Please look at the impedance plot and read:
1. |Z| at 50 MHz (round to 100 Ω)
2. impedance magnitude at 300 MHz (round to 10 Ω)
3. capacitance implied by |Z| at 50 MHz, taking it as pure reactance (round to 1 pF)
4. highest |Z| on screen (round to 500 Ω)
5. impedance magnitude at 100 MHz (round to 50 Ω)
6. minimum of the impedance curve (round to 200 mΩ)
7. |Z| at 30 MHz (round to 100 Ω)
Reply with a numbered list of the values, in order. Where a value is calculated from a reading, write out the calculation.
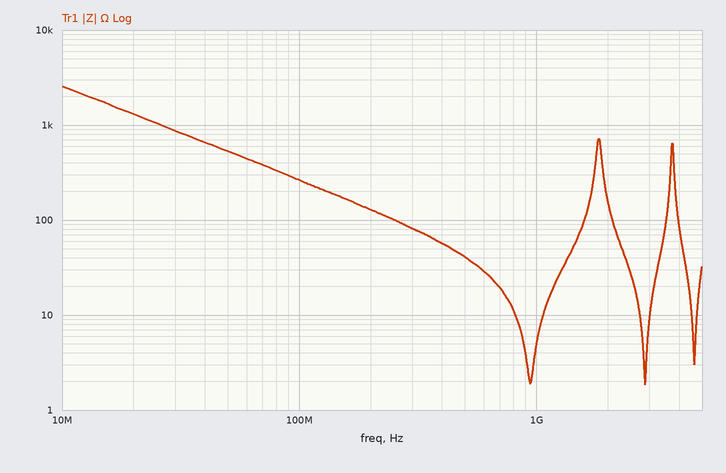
1. 500 Ω
2. 80 Ω
3. C = 1/(2π × 50 MHz × 500 Ω) ≈ 6 pF
4. 2.5 kΩ
5. 250 Ω
6. 1.8 Ω
7. 900 Ω
